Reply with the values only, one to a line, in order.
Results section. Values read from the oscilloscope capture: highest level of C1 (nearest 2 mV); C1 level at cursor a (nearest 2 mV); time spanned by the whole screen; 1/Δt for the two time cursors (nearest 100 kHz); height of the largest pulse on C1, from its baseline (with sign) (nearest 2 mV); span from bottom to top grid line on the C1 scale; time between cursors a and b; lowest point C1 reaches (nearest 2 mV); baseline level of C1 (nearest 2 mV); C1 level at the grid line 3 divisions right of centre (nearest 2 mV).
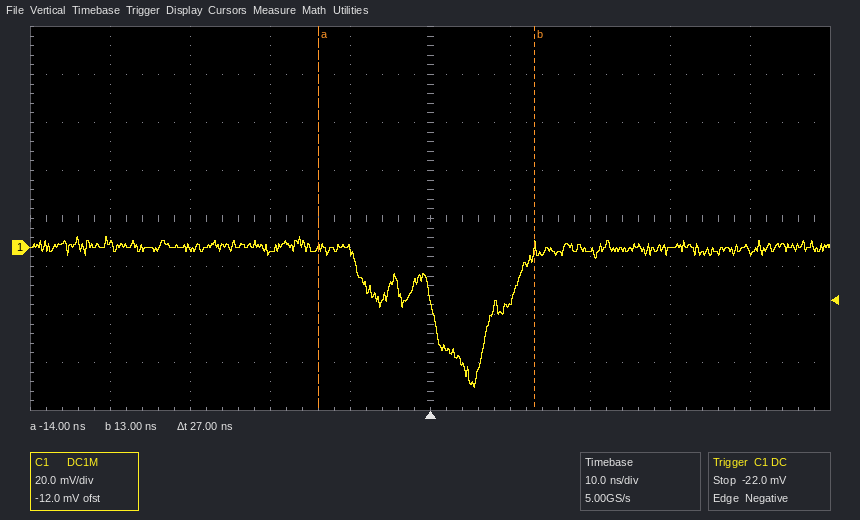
4 mV
0 mV
100 ns
37.0 MHz
-58 mV
160 mV
27 ns
-58 mV
0 mV
-2 mV
